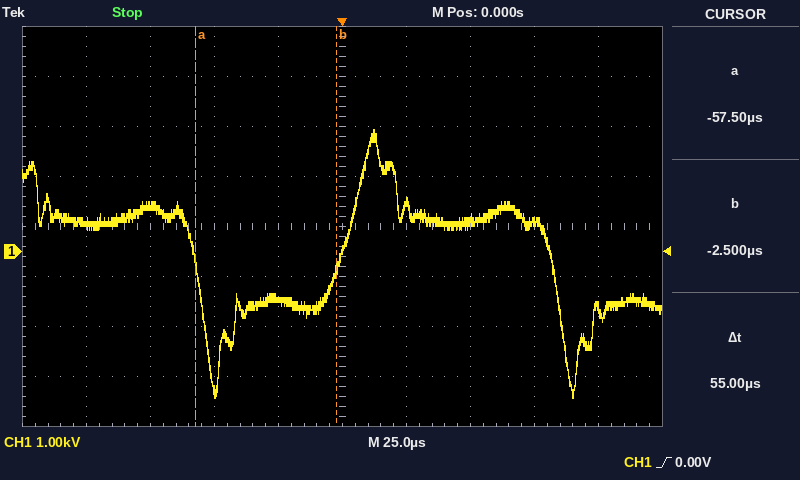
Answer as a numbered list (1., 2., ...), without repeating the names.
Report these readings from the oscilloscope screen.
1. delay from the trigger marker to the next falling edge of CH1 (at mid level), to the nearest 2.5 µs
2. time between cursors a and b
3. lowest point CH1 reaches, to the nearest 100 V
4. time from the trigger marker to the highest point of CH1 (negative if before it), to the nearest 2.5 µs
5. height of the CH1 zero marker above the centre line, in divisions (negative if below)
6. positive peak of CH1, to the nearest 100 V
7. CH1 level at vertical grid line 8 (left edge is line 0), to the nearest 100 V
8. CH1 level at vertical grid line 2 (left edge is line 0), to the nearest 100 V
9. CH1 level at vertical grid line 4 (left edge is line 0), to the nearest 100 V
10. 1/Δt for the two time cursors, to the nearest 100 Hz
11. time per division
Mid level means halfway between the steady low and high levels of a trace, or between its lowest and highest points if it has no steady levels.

1. 82.5 µs
2. 55 µs
3. -2.9 kV
4. +12.5 µs
5. -0.5 div
6. 2.4 kV
7. 600 V
8. 900 V
9. -900 V
10. 18.2 kHz
11. 25 µs
